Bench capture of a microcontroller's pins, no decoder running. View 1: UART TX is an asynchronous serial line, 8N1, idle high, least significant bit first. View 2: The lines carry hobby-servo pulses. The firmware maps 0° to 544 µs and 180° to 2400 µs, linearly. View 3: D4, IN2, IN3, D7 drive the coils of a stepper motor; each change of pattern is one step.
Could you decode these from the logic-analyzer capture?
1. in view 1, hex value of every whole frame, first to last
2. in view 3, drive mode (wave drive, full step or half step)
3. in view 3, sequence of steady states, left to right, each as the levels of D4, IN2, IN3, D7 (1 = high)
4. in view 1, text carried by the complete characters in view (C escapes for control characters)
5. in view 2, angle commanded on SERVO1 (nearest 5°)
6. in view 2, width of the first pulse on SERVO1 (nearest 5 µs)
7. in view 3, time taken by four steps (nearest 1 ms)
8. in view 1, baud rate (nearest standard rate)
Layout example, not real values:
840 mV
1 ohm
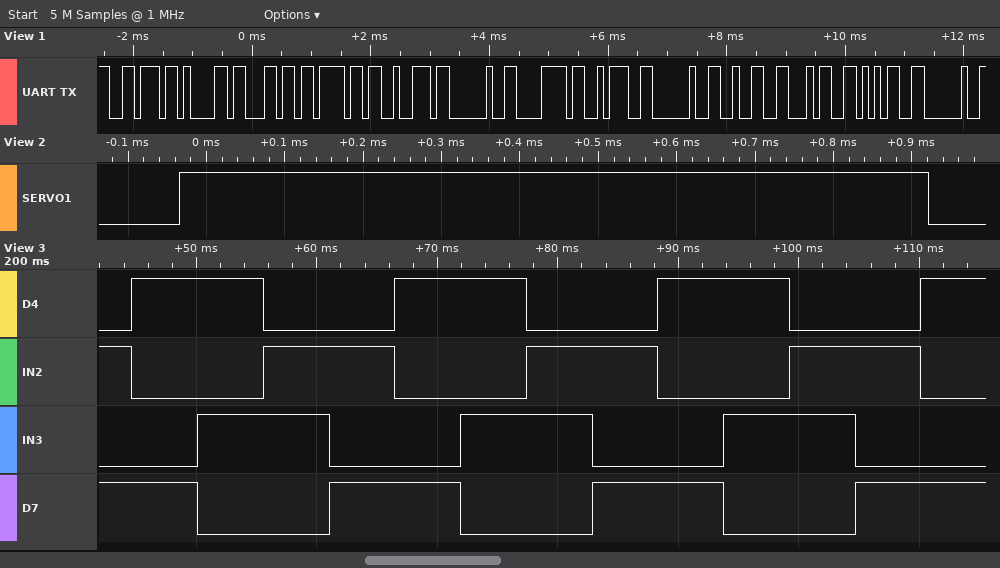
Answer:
76 61 6C 6F 72 20 78 3A 20 32 34 35 20
full step
0101 1001 1010 0110 0101 1001 1010 0110 0101 1001 1010 0110 0101 1001
"valor x: 245 "
40°
955 µs
22 ms
9600 baud
